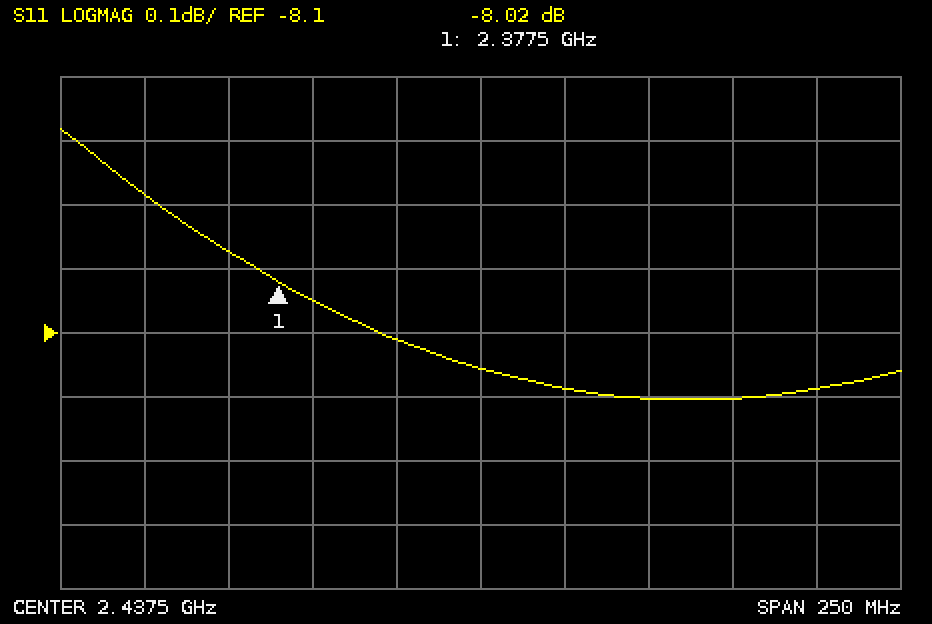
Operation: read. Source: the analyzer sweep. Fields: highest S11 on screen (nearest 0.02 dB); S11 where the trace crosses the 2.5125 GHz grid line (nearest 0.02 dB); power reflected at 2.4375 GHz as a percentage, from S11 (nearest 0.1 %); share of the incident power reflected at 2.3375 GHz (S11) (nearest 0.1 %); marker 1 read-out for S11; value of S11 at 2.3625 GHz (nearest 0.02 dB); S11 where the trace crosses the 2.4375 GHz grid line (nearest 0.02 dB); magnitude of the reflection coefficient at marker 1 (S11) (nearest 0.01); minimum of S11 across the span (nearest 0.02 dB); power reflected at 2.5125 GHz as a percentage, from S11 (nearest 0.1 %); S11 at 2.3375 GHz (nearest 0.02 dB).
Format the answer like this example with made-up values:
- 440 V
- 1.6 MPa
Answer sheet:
- -7.78 dB
- -8.20 dB
- 15.3 %
- 16.3 %
- -8.02 dB
- -7.98 dB
- -8.16 dB
- 0.40
- -8.20 dB
- 15.1 %
- -7.88 dB
